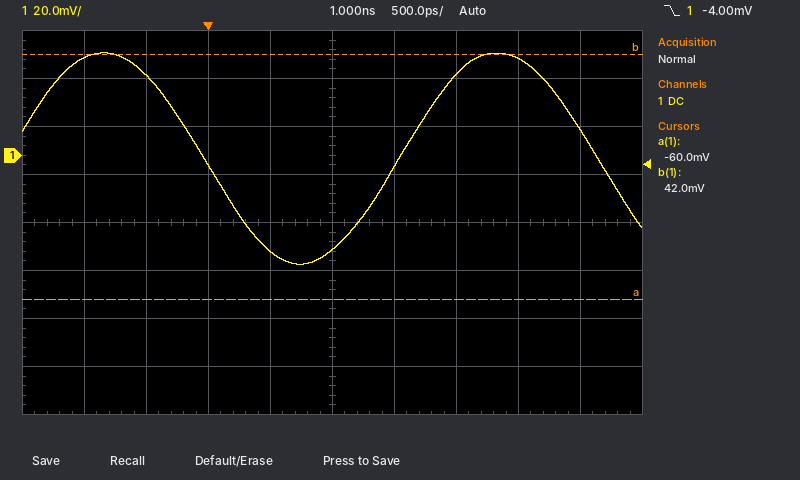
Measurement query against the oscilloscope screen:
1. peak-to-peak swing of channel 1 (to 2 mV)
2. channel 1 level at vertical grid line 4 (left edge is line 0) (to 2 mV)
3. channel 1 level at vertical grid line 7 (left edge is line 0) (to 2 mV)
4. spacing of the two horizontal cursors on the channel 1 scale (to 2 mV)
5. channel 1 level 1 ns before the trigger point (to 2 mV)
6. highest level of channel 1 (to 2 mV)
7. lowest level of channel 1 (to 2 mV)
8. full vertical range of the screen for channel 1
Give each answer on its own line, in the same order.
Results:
88 mV
-40 mV
34 mV
102 mV
40 mV
42 mV
-46 mV
160 mV
